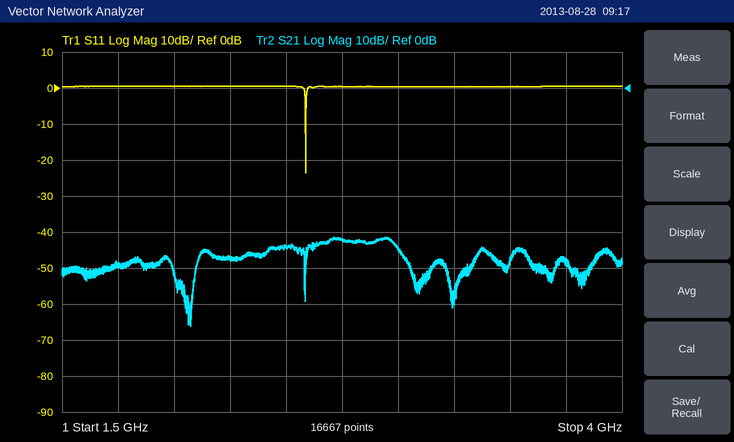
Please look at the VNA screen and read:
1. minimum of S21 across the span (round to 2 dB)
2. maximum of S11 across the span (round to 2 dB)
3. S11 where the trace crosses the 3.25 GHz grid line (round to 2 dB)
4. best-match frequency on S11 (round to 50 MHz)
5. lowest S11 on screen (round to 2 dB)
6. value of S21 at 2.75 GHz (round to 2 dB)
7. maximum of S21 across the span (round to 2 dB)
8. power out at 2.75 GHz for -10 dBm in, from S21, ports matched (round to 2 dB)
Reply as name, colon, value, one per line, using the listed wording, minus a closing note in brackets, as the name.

minimum of S21 across the span: -66 dB
maximum of S11 across the span: 0 dB
S11 where the trace crosses the 3.25 GHz grid line: 0 dB
best-match frequency on S11: 2.60 GHz
lowest S11 on screen: -24 dB
value of S21 at 2.75 GHz: -42 dB
maximum of S21 across the span: -42 dB
power out at 2.75 GHz for -10 dBm in, from S21, ports matched: -52 dBm
